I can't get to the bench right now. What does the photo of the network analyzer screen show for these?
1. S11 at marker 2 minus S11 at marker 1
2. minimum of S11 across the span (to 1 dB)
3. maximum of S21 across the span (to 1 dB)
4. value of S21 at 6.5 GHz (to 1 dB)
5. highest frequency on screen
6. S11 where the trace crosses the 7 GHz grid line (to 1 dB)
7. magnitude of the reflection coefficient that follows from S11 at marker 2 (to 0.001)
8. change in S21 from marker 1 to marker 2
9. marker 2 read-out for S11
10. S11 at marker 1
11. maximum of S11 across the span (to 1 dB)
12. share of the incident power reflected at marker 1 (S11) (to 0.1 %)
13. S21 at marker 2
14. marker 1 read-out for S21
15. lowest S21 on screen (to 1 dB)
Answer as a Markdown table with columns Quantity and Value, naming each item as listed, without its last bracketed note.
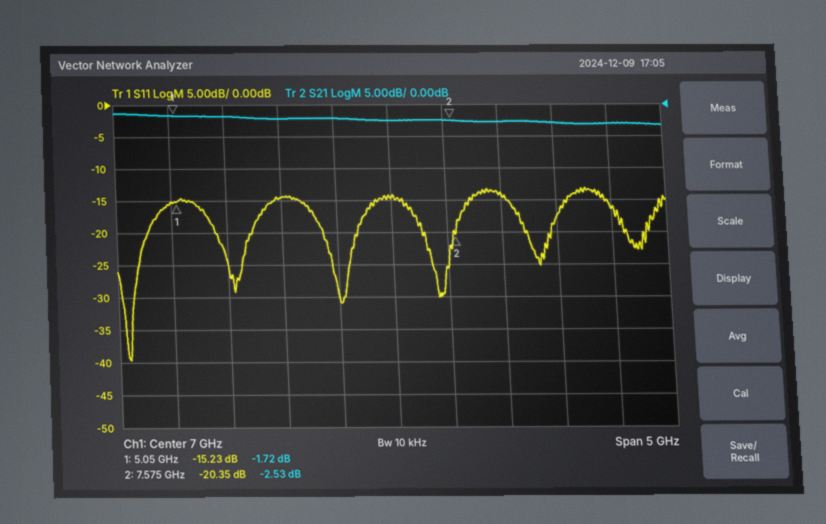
| Quantity | Value |
|---|---|
| S11 at marker 2 minus S11 at marker 1 | -5.12 dB |
| minimum of S11 across the span | -40 dB |
| maximum of S21 across the span | -1 dB |
| value of S21 at 6.5 GHz | -2 dB |
| highest frequency on screen | 9.5 GHz |
| S11 where the trace crosses the 7 GHz grid line | -15 dB |
| magnitude of the reflection coefficient that follows from S11 at marker 2 | 0.096 |
| change in S21 from marker 1 to marker 2 | -0.81 dB |
| marker 2 read-out for S11 | -20.35 dB |
| S11 at marker 1 | -15.23 dB |
| maximum of S11 across the span | -13 dB |
| share of the incident power reflected at marker 1 (S11) | 3.0 % |
| S21 at marker 2 | -2.53 dB |
| marker 1 read-out for S21 | -1.72 dB |
| lowest S21 on screen | -3 dB |
